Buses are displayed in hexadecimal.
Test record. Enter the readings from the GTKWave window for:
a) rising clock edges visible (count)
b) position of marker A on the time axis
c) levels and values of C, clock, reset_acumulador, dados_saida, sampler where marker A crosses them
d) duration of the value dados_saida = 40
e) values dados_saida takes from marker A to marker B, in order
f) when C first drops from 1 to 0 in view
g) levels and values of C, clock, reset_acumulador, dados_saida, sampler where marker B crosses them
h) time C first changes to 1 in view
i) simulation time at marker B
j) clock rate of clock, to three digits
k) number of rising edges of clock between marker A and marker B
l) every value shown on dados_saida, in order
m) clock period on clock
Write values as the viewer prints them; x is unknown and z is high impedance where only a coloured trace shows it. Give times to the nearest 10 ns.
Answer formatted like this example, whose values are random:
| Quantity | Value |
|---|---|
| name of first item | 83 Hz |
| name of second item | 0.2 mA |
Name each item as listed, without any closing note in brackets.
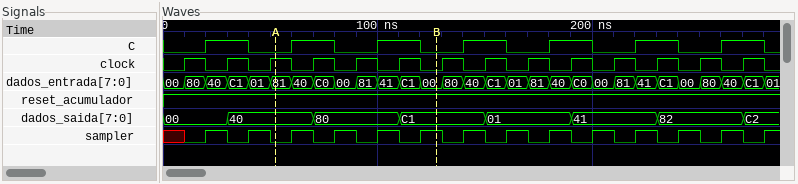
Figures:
| Quantity | Value |
|---|---|
| rising clock edges visible | 14 |
| position of marker A on the time axis | 50 ns |
| levels and values of C, clock, reset_acumulador, dados_saida, sampler where marker A crosses them | C=0, clock=1, reset_acumulador=1, dados_saida=40, sampler=0 |
| duration of the value dados_saida = 40 | 40 ns |
| values dados_saida takes from marker A to marker B, in order | 40, 80, C1 |
| when C first drops from 1 to 0 in view | 40 ns |
| levels and values of C, clock, reset_acumulador, dados_saida, sampler where marker B crosses them | C=0, clock=0, reset_acumulador=1, dados_saida=C1, sampler=1 |
| time C first changes to 1 in view | 20 ns |
| simulation time at marker B | 130 ns |
| clock rate of clock, to three digits | 50.0 MHz |
| number of rising edges of clock between marker A and marker B | 3 |
| every value shown on dados_saida, in order | 00, 40, 80, C1, 01, 41, 82, C2 |
| clock period on clock | 20 ns |
